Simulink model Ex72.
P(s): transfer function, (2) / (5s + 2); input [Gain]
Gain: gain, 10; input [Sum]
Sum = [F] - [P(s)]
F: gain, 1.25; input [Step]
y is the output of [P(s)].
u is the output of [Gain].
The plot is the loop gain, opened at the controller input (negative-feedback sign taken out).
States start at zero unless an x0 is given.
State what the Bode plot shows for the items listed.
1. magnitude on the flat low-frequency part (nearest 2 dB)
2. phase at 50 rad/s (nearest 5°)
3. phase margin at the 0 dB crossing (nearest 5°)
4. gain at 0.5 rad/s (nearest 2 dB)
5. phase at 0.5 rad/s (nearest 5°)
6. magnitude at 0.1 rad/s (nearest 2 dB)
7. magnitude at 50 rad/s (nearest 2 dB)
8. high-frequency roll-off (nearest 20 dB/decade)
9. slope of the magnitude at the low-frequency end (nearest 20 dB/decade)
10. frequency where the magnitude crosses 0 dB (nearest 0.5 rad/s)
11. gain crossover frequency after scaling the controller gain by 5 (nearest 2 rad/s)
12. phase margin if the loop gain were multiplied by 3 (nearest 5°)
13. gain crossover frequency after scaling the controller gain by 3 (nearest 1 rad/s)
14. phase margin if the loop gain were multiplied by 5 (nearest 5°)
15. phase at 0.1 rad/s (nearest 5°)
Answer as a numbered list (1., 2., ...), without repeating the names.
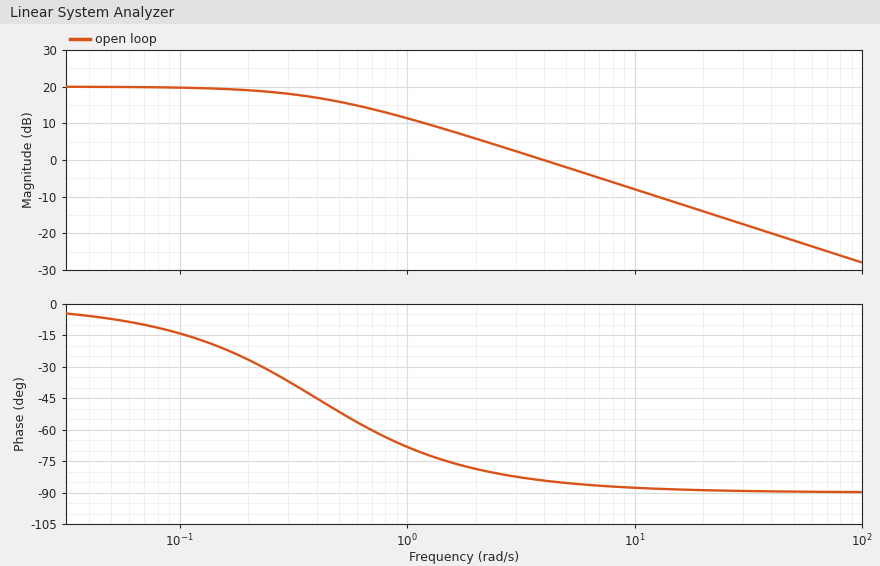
1. 20 dB
2. -90°
3. 95°
4. 16 dB
5. -50°
6. 20 dB
7. -22 dB
8. -20 dB/decade
9. 0 dB/decade
10. 4.0 rad/s
11. 20 rad/s
12. 90°
13. 12 rad/s
14. 90°
15. -15°
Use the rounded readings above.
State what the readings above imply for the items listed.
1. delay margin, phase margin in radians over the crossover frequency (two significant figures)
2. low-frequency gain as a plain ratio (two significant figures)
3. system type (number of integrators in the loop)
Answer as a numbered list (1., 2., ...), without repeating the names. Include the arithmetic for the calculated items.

1. 95 × π / 180 / 4 = 0.41 s
2. 10^(20 / 20) = 10
3. 0
